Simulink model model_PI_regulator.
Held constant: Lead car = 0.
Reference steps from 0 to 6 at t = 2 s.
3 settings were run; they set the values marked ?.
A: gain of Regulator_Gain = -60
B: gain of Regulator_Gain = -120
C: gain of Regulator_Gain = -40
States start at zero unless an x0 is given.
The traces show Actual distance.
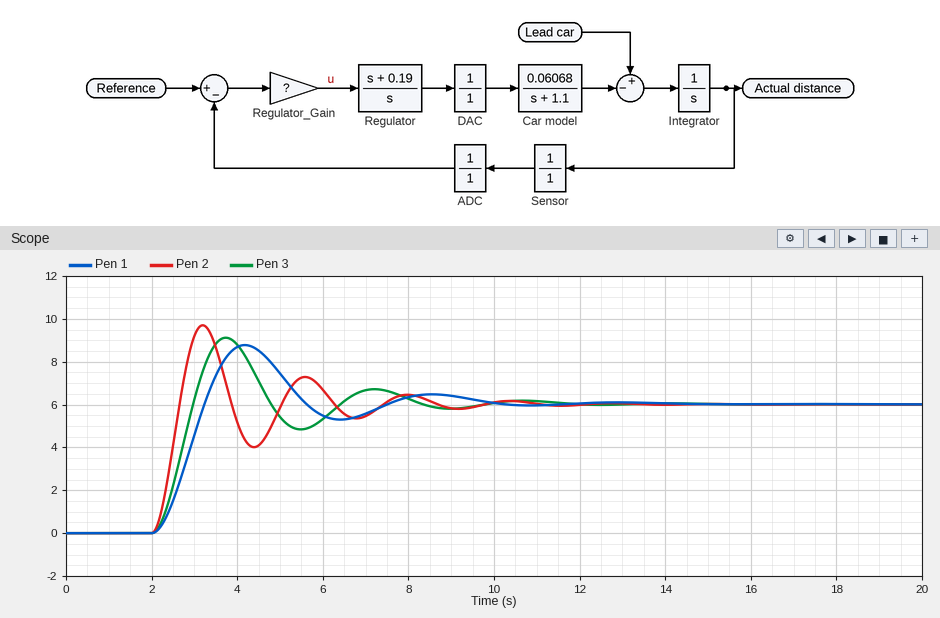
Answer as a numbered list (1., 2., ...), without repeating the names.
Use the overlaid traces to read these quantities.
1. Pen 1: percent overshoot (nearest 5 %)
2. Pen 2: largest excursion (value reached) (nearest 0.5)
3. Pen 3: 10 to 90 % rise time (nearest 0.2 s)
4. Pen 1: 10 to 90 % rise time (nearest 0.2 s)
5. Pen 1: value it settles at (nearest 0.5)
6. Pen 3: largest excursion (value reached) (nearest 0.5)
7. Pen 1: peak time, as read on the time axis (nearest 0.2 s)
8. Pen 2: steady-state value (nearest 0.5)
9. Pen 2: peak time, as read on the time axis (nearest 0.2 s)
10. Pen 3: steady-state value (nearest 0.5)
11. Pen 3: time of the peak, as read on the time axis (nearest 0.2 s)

1. 45 %
2. 9.5
3. 0.6 s
4. 0.8 s
5. 6.0
6. 9.0
7. 4.2 s
8. 6.0
9. 3.2 s
10. 6.0
11. 3.8 s
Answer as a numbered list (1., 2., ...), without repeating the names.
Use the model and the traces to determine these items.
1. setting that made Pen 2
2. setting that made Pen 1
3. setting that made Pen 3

1. B
2. C
3. A
